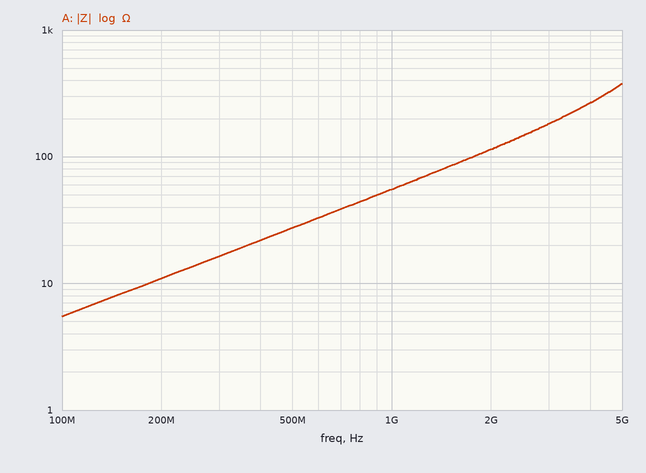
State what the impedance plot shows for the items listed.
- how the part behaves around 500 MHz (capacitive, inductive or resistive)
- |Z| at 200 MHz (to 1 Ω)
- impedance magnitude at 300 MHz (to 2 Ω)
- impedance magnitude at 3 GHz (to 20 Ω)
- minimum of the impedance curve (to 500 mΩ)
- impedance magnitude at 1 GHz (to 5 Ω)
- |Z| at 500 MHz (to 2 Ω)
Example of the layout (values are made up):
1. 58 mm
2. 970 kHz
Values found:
1. inductive
2. 11 Ω
3. 16 Ω
4. 180 Ω
5. 5.5 Ω
6. 55 Ω
7. 28 Ω
